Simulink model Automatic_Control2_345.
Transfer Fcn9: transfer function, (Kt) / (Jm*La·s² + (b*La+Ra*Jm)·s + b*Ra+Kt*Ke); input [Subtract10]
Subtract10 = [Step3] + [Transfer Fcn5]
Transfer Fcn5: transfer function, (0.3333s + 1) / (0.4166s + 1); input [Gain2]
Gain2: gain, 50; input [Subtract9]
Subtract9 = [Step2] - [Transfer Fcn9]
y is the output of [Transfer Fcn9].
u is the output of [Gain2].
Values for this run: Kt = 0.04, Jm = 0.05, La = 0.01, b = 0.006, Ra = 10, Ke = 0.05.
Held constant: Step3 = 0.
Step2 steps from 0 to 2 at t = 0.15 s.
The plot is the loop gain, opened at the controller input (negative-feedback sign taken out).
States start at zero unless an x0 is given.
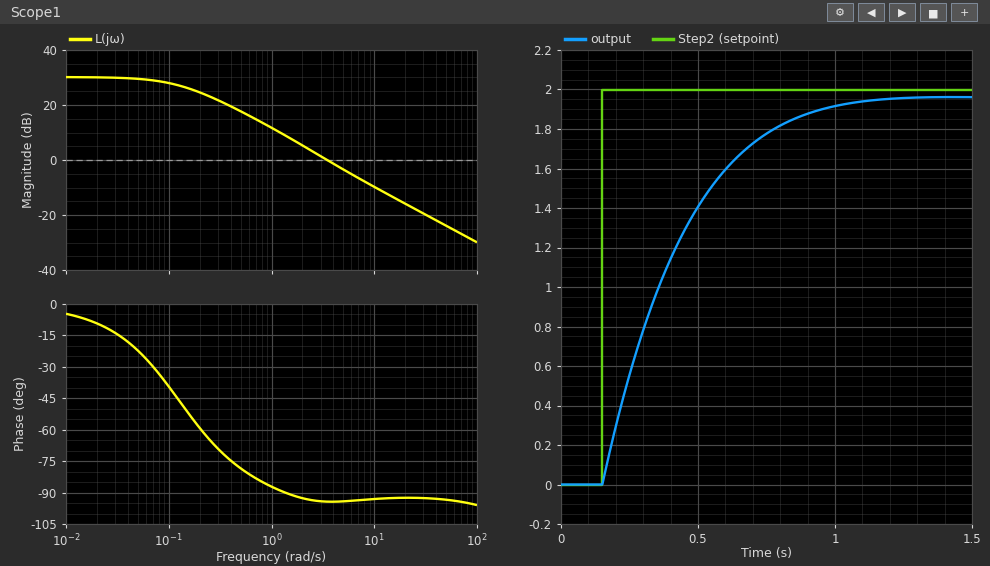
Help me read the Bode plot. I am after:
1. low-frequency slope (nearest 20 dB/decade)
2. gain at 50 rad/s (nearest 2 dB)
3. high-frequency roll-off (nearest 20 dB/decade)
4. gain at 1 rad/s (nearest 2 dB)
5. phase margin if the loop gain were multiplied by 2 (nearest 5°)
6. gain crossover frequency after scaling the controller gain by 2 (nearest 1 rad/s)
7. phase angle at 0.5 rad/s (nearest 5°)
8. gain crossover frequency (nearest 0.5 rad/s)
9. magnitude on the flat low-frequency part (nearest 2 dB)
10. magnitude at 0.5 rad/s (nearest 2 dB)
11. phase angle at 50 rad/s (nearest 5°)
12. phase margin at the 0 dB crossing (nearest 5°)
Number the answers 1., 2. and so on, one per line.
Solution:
1. 0 dB/decade
2. -24 dB
3. -20 dB/decade
4. 12 dB
5. 85°
6. 7 rad/s
7. -80°
8. 3.5 rad/s
9. 30 dB
10. 18 dB
11. -95°
12. 85°
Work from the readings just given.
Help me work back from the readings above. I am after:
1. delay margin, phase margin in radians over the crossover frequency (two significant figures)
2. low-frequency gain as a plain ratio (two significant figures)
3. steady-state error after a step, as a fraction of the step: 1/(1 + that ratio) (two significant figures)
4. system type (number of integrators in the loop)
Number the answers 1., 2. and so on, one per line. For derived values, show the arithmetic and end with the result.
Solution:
1. 85 × π / 180 / 3.5 = 0.42 s
2. 10^(30 / 20) = 32
3. 1 / (1 + 32) = 0.030
4. 0
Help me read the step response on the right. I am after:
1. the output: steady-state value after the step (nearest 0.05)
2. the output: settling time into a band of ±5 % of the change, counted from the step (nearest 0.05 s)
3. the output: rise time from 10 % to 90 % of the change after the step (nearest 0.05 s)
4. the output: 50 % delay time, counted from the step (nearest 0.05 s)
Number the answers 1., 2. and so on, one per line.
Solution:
1. 1.95
2. 0.70 s
3. 0.55 s
4. 0.20 s
